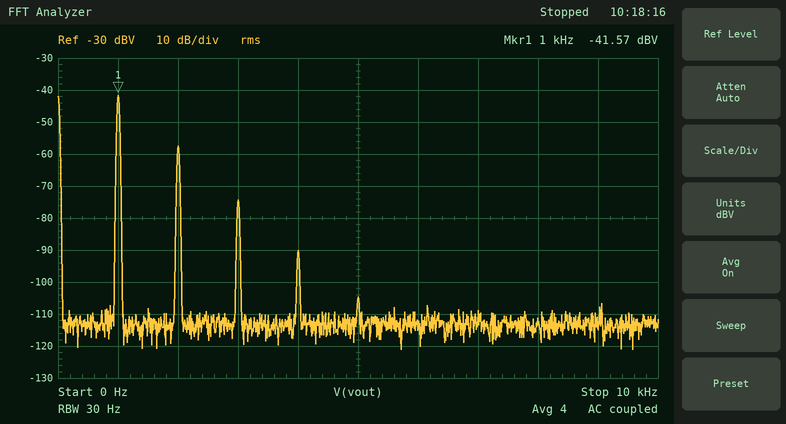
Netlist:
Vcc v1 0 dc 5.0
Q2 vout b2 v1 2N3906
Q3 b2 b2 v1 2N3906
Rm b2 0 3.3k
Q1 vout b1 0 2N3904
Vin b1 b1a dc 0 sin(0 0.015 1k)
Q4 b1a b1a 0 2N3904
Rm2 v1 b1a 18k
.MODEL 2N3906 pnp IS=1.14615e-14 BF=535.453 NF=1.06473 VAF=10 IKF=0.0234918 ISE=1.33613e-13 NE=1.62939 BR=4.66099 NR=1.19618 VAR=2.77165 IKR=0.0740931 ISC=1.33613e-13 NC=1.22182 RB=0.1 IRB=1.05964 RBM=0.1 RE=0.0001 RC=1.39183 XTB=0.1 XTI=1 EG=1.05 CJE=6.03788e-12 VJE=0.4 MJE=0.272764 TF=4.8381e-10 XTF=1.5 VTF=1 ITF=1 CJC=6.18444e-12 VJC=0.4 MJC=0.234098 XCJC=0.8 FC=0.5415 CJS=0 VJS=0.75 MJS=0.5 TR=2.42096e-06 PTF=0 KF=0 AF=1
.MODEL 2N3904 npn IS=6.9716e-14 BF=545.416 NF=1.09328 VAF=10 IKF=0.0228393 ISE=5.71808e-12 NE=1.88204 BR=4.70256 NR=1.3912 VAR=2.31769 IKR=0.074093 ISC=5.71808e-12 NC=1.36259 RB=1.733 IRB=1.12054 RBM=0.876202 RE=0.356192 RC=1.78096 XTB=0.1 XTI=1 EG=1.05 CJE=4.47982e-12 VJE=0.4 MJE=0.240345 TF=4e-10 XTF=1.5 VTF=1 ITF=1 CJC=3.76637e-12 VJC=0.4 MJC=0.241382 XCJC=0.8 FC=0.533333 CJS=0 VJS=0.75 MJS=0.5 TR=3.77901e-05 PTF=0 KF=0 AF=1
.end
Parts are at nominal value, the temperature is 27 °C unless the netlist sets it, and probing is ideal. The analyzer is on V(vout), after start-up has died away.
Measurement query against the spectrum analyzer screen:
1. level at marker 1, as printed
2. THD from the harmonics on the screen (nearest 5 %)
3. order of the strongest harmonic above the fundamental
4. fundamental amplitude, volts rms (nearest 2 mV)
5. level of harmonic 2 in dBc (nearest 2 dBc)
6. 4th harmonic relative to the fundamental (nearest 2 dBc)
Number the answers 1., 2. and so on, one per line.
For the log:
1. -41.57 dBV
2. 15 %
3. 2
4. 8 mV
5. -16 dBc
6. -48 dBc
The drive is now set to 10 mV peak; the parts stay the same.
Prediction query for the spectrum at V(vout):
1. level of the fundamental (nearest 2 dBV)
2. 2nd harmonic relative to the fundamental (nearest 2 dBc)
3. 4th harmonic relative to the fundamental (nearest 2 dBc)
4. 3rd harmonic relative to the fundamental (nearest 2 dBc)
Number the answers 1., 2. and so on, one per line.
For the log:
1. -46 dBV
2. -20 dBc
3. -60 dBc
4. -40 dBc
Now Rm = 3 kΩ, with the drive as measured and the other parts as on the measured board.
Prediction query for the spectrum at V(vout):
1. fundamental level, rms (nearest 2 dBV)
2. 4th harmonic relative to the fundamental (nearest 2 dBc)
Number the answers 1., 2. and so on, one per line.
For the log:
1. -42 dBV
2. -50 dBc
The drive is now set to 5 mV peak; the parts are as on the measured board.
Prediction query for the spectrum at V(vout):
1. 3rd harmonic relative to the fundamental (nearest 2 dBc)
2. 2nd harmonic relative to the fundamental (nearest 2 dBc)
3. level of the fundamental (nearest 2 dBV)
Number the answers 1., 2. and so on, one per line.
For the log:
1. -52 dBc
2. -26 dBc
3. -52 dBV
